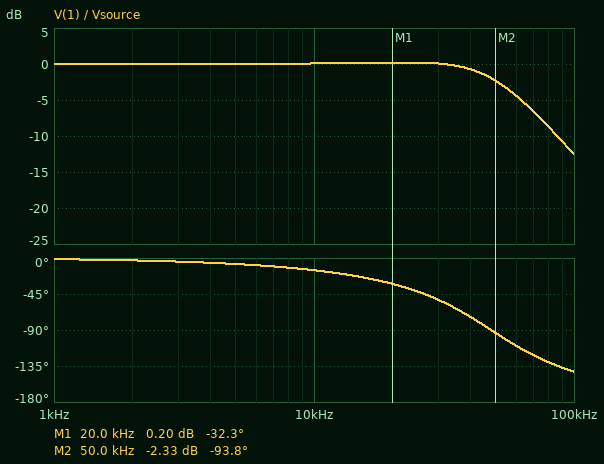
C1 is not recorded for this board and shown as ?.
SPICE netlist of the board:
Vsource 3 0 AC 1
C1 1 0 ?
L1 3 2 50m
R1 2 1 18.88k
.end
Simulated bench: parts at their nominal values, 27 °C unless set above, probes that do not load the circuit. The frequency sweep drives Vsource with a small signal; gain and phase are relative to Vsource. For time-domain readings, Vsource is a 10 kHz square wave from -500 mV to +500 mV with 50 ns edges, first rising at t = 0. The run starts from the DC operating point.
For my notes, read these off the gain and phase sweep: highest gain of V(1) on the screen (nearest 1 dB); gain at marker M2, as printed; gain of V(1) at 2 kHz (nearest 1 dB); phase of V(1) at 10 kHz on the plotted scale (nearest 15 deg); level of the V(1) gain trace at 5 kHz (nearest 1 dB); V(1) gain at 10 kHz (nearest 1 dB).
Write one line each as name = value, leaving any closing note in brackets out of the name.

highest gain of V(1) on the screen = 0 dB
gain at marker M2, as printed = -2.33 dB
gain of V(1) at 2 kHz = 0 dB
phase of V(1) at 10 kHz on the plotted scale = -15 deg
level of the V(1) gain trace at 5 kHz = 0 dB
V(1) gain at 10 kHz = 0 dB
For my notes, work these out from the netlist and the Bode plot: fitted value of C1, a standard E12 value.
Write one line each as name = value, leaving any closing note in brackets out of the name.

fitted value of C1, a standard E12 value = 220 pF
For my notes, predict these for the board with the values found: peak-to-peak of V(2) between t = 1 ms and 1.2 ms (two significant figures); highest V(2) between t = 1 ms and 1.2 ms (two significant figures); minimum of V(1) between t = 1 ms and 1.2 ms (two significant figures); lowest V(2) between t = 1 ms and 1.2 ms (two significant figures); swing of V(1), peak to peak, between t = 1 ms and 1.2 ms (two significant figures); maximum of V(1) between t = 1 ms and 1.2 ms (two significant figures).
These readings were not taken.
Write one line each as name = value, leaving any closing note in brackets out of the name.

peak-to-peak of V(2) between t = 1 ms and 1.2 ms = 1.5 V
highest V(2) between t = 1 ms and 1.2 ms = 740 mV
minimum of V(1) between t = 1 ms and 1.2 ms = -580 mV
lowest V(2) between t = 1 ms and 1.2 ms = -740 mV
swing of V(1), peak to peak, between t = 1 ms and 1.2 ms = 1.2 V
maximum of V(1) between t = 1 ms and 1.2 ms = 580 mV
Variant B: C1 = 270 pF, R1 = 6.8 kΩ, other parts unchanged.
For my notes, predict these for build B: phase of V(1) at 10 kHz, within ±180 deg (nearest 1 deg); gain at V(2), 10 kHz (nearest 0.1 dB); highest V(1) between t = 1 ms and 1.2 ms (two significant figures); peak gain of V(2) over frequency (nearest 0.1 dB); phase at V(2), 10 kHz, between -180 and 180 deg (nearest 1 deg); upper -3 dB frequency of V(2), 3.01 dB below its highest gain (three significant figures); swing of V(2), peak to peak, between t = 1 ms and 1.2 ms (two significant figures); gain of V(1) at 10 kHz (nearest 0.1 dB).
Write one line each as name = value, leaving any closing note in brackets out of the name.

phase of V(1) at 10 kHz, within ±180 deg = -7 deg
gain at V(2), 10 kHz = 0.5 dB
highest V(1) between t = 1 ms and 1.2 ms = 930 mV
peak gain of V(2) over frequency = 7.2 dB
phase at V(2), 10 kHz, between -180 and 180 deg = 0 deg
upper -3 dB frequency of V(2), 3.01 dB below its highest gain = 51.4 kHz
swing of V(2), peak to peak, between t = 1 ms and 1.2 ms = 2.0 V
gain of V(1) at 10 kHz = 0.4 dB
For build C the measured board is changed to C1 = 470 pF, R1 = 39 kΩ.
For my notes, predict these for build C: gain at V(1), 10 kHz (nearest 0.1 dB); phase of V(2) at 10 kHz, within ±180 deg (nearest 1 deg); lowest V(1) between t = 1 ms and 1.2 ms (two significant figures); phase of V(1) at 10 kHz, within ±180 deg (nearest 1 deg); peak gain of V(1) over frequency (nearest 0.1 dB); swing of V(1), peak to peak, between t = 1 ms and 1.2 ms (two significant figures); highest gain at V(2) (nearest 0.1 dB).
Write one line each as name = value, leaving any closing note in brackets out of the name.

gain at V(1), 10 kHz = -3.3 dB
phase of V(2) at 10 kHz, within ±180 deg = -3 deg
lowest V(1) between t = 1 ms and 1.2 ms = -450 mV
phase of V(1) at 10 kHz, within ±180 deg = -52 deg
peak gain of V(1) over frequency = 0 dB
swing of V(1), peak to peak, between t = 1 ms and 1.2 ms = 890 mV
highest gain at V(2) = 0.4 dB
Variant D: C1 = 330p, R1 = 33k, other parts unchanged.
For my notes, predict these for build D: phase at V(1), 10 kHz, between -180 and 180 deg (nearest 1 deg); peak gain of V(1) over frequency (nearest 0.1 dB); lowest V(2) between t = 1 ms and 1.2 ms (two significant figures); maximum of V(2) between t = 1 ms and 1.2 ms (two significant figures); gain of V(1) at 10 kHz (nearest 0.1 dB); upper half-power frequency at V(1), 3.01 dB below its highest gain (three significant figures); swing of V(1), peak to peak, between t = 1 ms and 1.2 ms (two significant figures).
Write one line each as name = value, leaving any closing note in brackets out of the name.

phase at V(1), 10 kHz, between -180 and 180 deg = -36 deg
peak gain of V(1) over frequency = 0 dB
lowest V(2) between t = 1 ms and 1.2 ms = -590 mV
maximum of V(2) between t = 1 ms and 1.2 ms = 590 mV
gain of V(1) at 10 kHz = -1.3 dB
upper half-power frequency at V(1), 3.01 dB below its highest gain = 16.9 kHz
swing of V(1), peak to peak, between t = 1 ms and 1.2 ms = 990 mV
